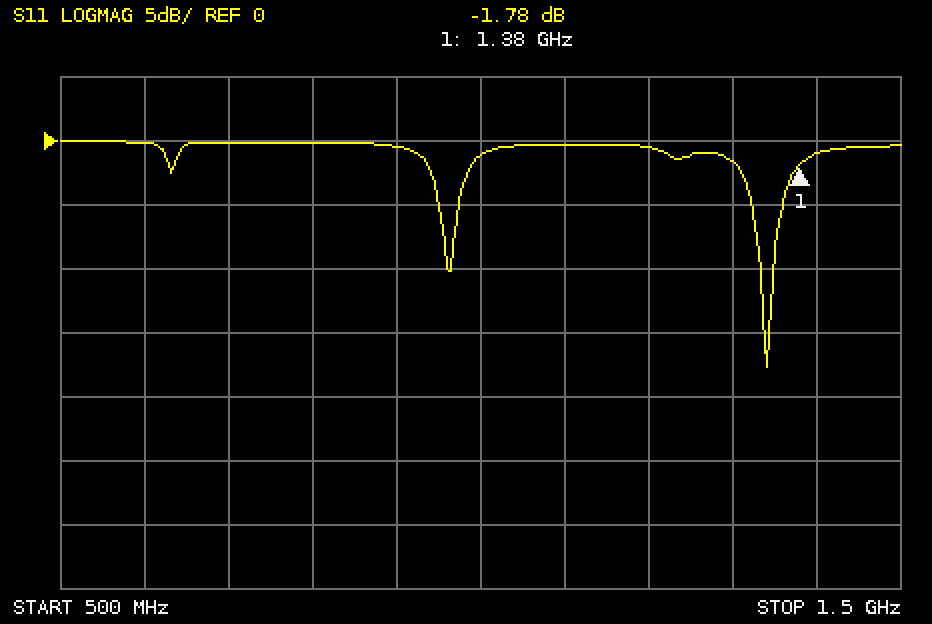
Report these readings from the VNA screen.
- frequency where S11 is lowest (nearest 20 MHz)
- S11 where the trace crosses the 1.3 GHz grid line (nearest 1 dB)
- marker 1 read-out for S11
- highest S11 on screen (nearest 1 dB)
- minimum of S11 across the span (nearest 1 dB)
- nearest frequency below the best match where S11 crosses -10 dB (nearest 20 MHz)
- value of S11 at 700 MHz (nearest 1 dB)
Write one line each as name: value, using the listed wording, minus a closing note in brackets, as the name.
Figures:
frequency where S11 is lowest: 1.34 GHz
S11 where the trace crosses the 1.3 GHz grid line: -2 dB
marker 1 read-out for S11: -1.78 dB
highest S11 on screen: 0 dB
minimum of S11 across the span: -18 dB
nearest frequency below the best match where S11 crosses -10 dB: 1.34 GHz
value of S11 at 700 MHz: 0 dB
